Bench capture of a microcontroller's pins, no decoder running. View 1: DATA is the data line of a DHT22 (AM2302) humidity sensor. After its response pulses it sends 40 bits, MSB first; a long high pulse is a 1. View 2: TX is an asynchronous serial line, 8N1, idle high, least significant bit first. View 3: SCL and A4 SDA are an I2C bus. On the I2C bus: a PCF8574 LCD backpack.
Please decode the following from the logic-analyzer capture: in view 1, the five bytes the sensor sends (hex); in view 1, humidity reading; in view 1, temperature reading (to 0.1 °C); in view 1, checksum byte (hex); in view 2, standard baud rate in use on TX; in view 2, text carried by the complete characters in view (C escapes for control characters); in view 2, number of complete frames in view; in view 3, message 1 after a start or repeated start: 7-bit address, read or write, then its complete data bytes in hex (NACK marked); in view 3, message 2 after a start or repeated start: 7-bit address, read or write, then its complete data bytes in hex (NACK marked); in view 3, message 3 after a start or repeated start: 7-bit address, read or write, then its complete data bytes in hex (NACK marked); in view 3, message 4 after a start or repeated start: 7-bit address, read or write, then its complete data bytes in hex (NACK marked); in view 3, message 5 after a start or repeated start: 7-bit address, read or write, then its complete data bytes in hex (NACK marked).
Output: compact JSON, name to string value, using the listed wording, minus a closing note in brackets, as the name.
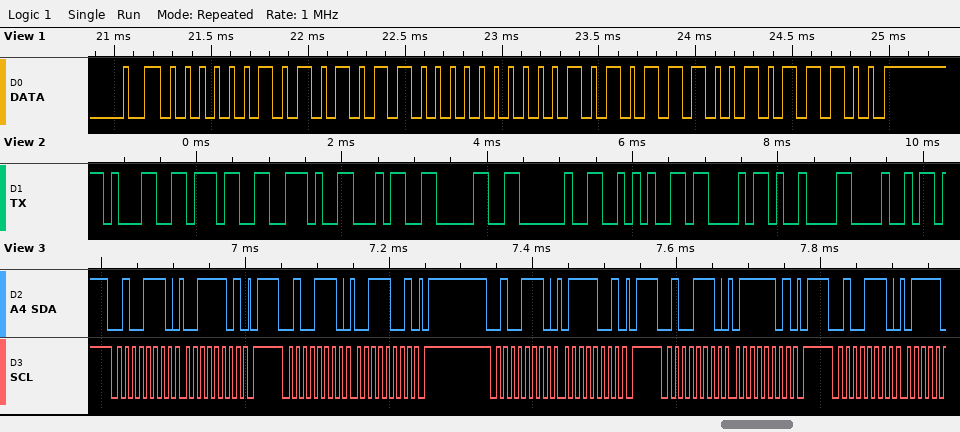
{"in view 1, the five bytes the sensor sends": "02 AC 00 AE 5C", "in view 1, humidity reading": "68.4 %", "in view 1, temperature reading": "17.4 °C", "in view 1, checksum byte": "0x5C", "in view 2, standard baud rate in use on TX": "9600 baud", "in view 2, text carried by the complete characters in view": "\"17.40 *C\\tH\"", "in view 2, number of complete frames in view": "10", "in view 3, message 1 after a start or repeated start: 7-bit address, read or write, then its complete data bytes in hex": "0x27 write: 3D", "in view 3, message 2 after a start or repeated start: 7-bit address, read or write, then its complete data bytes in hex": "0x27 write: 39", "in view 3, message 3 after a start or repeated start: 7-bit address, read or write, then its complete data bytes in hex": "0x27 write: 79", "in view 3, message 4 after a start or repeated start: 7-bit address, read or write, then its complete data bytes in hex": "0x27 write: 7D", "in view 3, message 5 after a start or repeated start: 7-bit address, read or write, then its complete data bytes in hex": "0x27 write"}
